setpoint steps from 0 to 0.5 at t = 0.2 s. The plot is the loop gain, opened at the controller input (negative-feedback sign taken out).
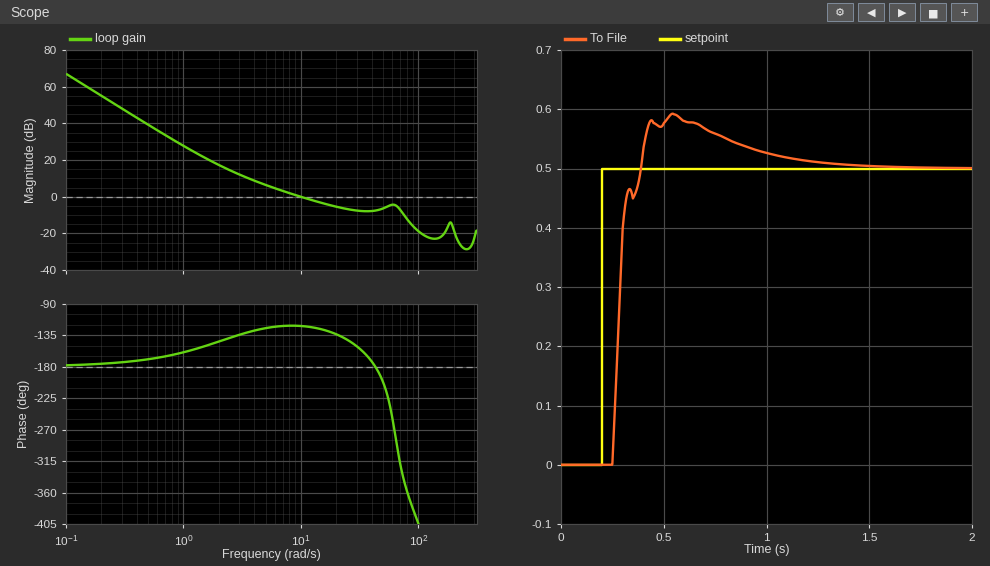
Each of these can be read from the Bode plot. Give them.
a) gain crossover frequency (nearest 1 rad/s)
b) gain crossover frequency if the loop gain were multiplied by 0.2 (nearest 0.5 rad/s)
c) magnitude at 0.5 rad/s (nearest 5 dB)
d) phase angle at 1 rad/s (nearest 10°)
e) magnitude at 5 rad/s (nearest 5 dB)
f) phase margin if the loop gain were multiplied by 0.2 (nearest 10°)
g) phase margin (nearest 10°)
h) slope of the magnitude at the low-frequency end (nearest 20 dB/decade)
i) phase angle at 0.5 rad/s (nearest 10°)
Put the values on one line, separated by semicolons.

10 rad/s; 2.5 rad/s; 40 dB; -160°; 5 dB; 40°; 60°; -40 dB/decade; -170°
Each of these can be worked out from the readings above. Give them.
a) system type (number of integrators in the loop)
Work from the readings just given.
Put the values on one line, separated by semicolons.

2
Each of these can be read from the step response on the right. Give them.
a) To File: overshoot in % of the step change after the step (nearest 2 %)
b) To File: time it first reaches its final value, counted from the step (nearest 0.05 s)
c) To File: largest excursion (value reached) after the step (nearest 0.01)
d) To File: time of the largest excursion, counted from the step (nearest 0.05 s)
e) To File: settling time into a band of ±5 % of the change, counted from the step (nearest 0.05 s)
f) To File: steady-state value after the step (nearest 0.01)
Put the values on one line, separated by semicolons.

18 %; 0.20 s; 0.59; 0.35 s; 0.80 s; 0.50
